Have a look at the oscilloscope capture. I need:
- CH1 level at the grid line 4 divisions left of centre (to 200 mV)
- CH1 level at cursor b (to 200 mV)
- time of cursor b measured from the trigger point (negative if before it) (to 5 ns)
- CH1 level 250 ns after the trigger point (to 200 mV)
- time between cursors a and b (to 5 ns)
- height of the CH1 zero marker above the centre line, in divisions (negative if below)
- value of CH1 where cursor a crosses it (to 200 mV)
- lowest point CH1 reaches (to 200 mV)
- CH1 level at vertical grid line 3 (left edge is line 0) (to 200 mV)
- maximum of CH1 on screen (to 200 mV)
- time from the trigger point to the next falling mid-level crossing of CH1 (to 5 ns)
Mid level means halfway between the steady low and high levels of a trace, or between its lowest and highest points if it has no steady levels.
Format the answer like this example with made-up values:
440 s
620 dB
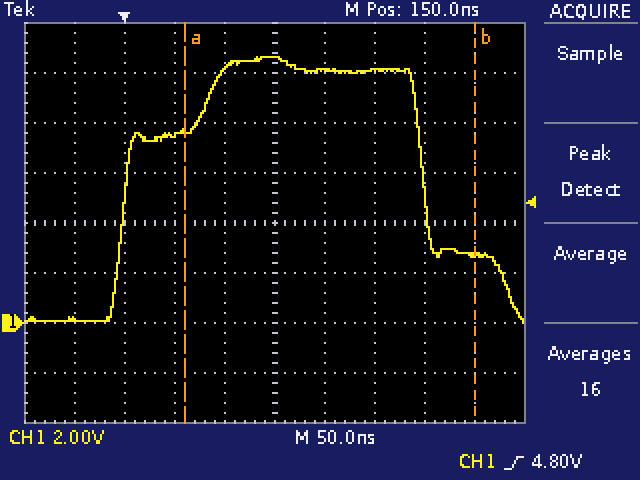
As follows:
200 mV
2.8 V
+350 ns
10.2 V
290 ns
-2.0 div
7.6 V
0.0 V
7.6 V
10.6 V
300 ns
